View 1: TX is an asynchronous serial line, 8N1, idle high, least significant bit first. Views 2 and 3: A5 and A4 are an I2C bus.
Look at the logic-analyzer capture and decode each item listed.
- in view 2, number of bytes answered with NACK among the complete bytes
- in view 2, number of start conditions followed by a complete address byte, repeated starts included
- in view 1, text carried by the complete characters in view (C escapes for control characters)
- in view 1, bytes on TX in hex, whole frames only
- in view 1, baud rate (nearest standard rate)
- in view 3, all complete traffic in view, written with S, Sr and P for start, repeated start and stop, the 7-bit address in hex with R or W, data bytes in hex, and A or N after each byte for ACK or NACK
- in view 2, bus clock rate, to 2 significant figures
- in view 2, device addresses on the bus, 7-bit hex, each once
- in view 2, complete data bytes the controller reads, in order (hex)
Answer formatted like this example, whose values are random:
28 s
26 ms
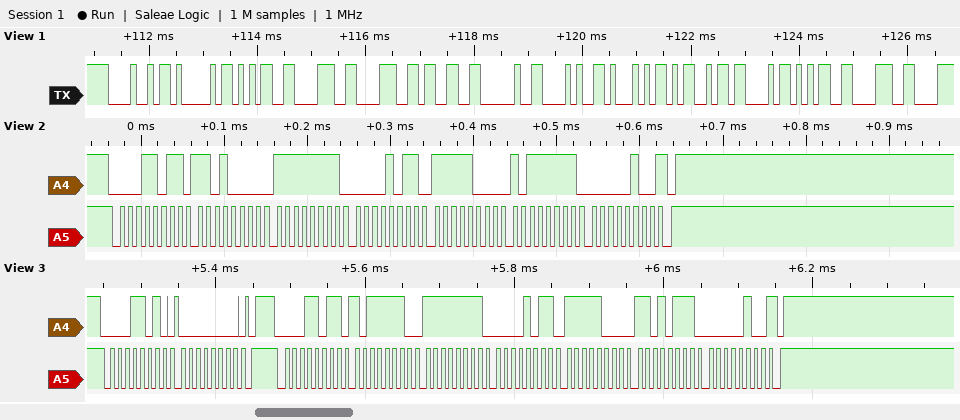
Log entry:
1
1
"HA5883 (QMC58"
48 41 35 38 38 33 20 28 51 4D 43 35 38
9600 baud
S 0DW A 00 A P S 0DR A BE A FF A 0B A F8 A D7 A 04 N P
100 kHz
0x0D
D0 FF 0B F8 BF 04
